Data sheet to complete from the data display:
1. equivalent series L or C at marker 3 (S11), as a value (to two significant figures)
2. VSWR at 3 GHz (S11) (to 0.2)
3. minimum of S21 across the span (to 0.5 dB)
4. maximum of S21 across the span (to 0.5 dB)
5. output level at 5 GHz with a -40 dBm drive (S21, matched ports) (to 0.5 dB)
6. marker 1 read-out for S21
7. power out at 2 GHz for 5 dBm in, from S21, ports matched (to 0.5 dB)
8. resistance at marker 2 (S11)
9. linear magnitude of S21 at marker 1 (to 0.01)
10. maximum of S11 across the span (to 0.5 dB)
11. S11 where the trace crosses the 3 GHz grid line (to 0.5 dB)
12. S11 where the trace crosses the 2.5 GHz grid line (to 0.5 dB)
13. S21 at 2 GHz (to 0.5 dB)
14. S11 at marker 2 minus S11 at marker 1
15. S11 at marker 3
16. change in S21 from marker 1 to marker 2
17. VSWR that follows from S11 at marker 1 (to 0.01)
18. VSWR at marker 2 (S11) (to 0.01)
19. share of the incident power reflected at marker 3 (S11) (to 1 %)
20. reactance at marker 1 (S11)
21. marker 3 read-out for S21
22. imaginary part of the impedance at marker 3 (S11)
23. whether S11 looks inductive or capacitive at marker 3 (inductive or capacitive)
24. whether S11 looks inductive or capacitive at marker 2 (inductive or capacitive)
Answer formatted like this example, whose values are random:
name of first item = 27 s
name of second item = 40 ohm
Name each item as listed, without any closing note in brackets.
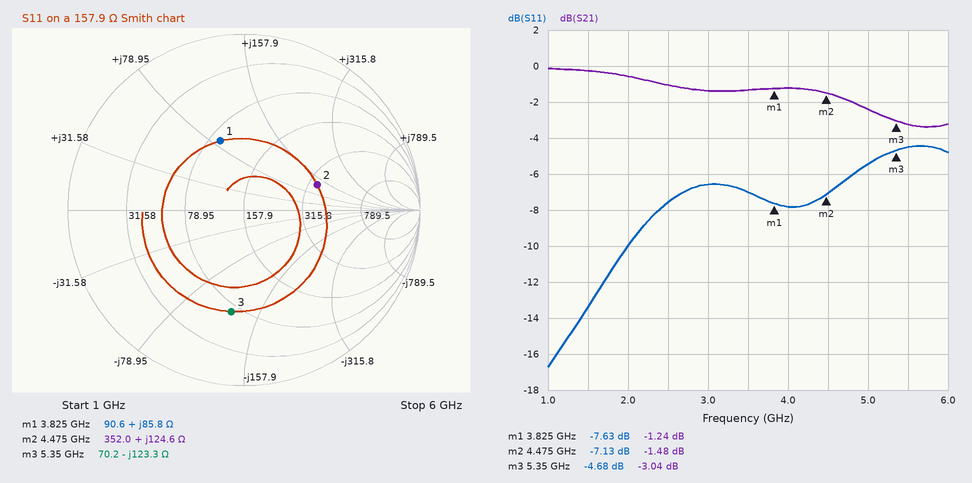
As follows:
equivalent series L or C at marker 3 (S11), as a value = 240 fF
VSWR at 3 GHz (S11) = 2.8
minimum of S21 across the span = -3.5 dB
maximum of S21 across the span = 0.0 dB
output level at 5 GHz with a -40 dBm drive (S21, matched ports) = -42.5 dBm
marker 1 read-out for S21 = -1.24 dB
power out at 2 GHz for 5 dBm in, from S21, ports matched = 4.5 dBm
resistance at marker 2 = 352.0 Ω
linear magnitude of S21 at marker 1 = 0.87
maximum of S11 across the span = -4.5 dB
S11 where the trace crosses the 3 GHz grid line = -6.5 dB
S11 where the trace crosses the 2.5 GHz grid line = -7.5 dB
S21 at 2 GHz = -0.5 dB
S11 at marker 2 minus S11 at marker 1 = 0.50 dB
S11 at marker 3 = -4.68 dB
change in S21 from marker 1 to marker 2 = -0.24 dB
VSWR that follows from S11 at marker 1 = 2.42
VSWR at marker 2 (S11) = 2.57
share of the incident power reflected at marker 3 (S11) = 34 %
reactance at marker 1 = +85.8 Ω
marker 3 read-out for S21 = -3.04 dB
imaginary part of the impedance at marker 3 = -123.3 Ω
whether S11 looks inductive or capacitive at marker 3 = capacitive
whether S11 looks inductive or capacitive at marker 2 = inductive
